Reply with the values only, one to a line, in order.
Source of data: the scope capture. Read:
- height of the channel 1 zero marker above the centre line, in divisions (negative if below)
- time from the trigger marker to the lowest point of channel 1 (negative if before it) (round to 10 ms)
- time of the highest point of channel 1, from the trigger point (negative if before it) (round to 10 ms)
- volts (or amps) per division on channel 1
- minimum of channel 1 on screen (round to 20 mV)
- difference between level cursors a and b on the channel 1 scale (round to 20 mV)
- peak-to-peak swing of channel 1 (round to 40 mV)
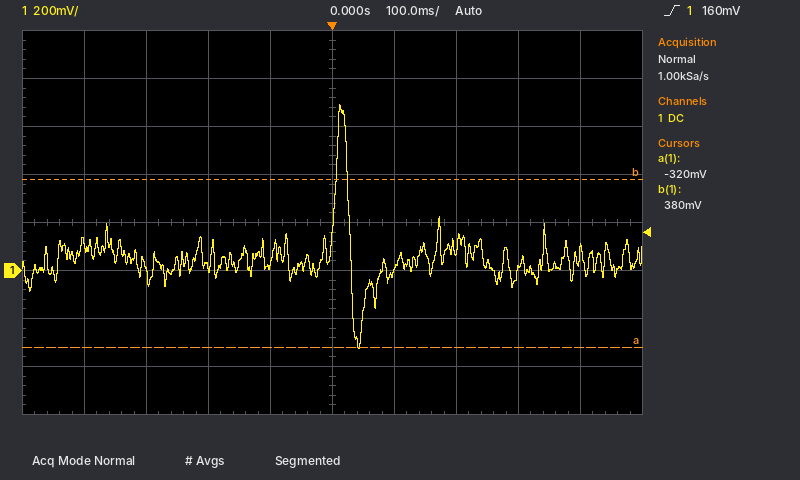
-1.0 div
+40 ms
+10 ms
200 mV
-320 mV
700 mV
1.00 V
